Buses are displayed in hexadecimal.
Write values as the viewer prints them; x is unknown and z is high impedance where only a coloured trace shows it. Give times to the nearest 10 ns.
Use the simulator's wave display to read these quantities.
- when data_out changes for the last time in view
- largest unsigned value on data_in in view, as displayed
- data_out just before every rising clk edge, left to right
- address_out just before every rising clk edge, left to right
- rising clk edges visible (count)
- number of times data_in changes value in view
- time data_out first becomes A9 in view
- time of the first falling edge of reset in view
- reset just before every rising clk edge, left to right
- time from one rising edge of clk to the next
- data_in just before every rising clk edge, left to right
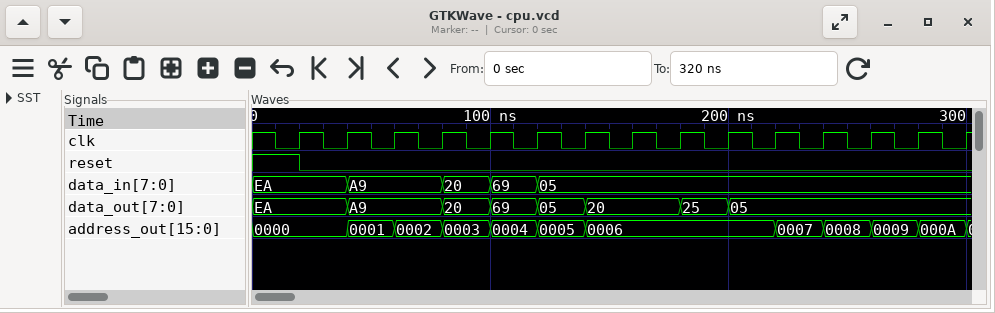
200 ns
EA
EA, EA, A9, A9, 20, 69, 05, 20, 20, 25, 05, 05, 05, 05, 05
0000, 0000, 0001, 0002, 0003, 0004, 0005, 0006, 0006, 0006, 0006, 0007, 0008, 0009, 000A
15
4
40 ns
20 ns
1 0 0 0 0 0 0 0 0 0 0 0 0 0 0
20 ns
EA, EA, A9, A9, 20, 69, 05, 05, 05, 05, 05, 05, 05, 05, 05
